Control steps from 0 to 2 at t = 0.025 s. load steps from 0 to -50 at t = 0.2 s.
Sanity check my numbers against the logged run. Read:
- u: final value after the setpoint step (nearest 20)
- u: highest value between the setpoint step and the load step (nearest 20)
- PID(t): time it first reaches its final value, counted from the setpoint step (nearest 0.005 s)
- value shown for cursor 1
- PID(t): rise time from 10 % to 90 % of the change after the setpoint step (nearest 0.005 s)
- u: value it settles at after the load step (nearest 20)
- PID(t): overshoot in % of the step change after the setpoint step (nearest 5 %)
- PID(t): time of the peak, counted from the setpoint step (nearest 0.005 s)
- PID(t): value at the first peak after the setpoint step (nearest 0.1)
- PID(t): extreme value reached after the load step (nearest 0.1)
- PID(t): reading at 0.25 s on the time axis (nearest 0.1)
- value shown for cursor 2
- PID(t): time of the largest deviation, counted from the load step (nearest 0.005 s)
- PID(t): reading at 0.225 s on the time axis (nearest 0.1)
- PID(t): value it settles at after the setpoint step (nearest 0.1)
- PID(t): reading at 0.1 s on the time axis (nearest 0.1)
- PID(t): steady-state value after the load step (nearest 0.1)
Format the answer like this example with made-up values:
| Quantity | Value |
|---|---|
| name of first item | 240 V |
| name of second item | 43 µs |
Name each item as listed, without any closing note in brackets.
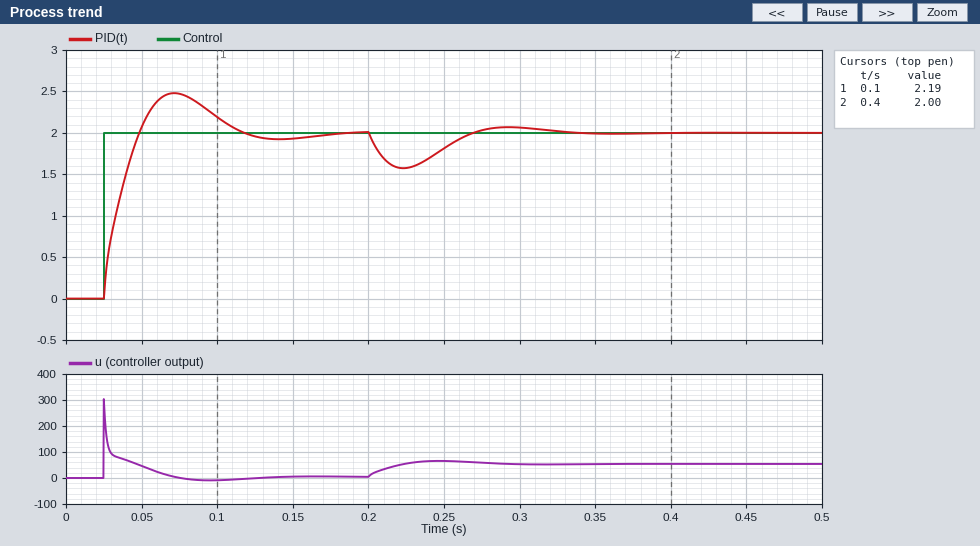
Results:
| Quantity | Value |
|---|---|
| u: final value after the setpoint step | 0 |
| u: highest value between the setpoint step and the load step | 300 |
| PID(t): time it first reaches its final value, counted from the setpoint step | 0.025 s |
| value shown for cursor 1 | 2.19 |
| PID(t): rise time from 10 % to 90 % of the change after the setpoint step | 0.020 s |
| u: value it settles at after the load step | 60 |
| PID(t): overshoot in % of the step change after the setpoint step | 25 % |
| PID(t): time of the peak, counted from the setpoint step | 0.045 s |
| PID(t): value at the first peak after the setpoint step | 2.5 |
| PID(t): extreme value reached after the load step | 1.6 |
| PID(t): reading at 0.25 s on the time axis | 1.8 |
| value shown for cursor 2 | 2.00 |
| PID(t): time of the largest deviation, counted from the load step | 0.025 s |
| PID(t): reading at 0.225 s on the time axis | 1.6 |
| PID(t): value it settles at after the setpoint step | 2.0 |
| PID(t): reading at 0.1 s on the time axis | 2.2 |
| PID(t): steady-state value after the load step | 2.0 |
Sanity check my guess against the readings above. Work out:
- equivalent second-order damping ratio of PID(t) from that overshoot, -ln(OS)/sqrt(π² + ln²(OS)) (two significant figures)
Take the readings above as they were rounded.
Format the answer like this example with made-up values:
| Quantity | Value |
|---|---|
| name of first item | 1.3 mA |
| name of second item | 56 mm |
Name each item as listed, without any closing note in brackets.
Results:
| Quantity | Value |
|---|---|
| equivalent second-order damping ratio of PID(t) from that overshoot, -ln(OS)/sqrt(π² + ln²(OS)) | 0.40 |
